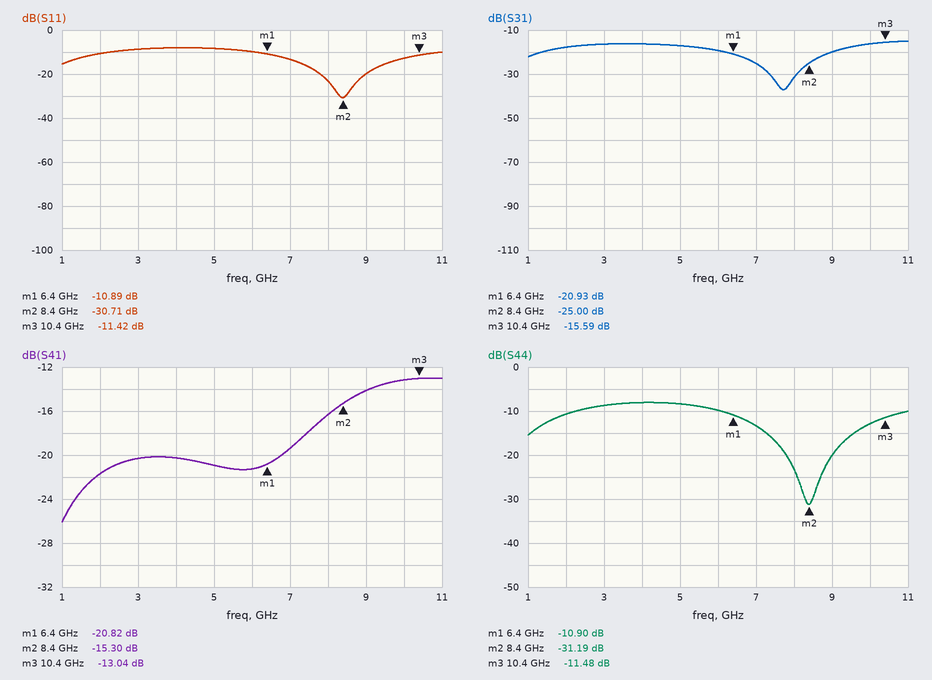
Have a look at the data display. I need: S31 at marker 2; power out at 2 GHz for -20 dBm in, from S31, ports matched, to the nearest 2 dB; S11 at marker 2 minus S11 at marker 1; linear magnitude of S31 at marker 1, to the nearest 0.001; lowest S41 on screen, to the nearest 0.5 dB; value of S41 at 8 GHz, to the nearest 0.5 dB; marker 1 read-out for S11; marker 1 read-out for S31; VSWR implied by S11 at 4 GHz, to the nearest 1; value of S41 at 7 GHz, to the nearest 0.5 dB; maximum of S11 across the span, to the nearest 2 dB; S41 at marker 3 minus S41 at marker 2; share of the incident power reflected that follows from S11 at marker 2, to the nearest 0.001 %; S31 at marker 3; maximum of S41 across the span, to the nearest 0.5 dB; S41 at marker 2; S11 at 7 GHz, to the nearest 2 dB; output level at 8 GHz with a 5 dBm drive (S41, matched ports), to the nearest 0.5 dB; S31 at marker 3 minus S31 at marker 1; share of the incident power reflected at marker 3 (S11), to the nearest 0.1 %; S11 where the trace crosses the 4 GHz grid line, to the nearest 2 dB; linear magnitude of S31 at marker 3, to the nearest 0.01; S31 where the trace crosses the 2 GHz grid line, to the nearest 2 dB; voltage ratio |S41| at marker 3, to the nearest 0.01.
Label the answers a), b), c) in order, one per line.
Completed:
a) -25.00 dB
b) -38 dBm
c) -19.82 dB
d) 0.090
e) -26.0 dB
f) -16.5 dB
g) -10.89 dB
h) -20.93 dB
i) 2
j) -19.5 dB
k) -8 dB
l) 2.26 dB
m) 0.085 %
n) -15.59 dB
o) -13.0 dB
p) -15.30 dB
q) -14 dB
r) -11.5 dBm
s) 5.34 dB
t) 7.2 %
u) -8 dB
v) 0.17
w) -18 dB
x) 0.22
